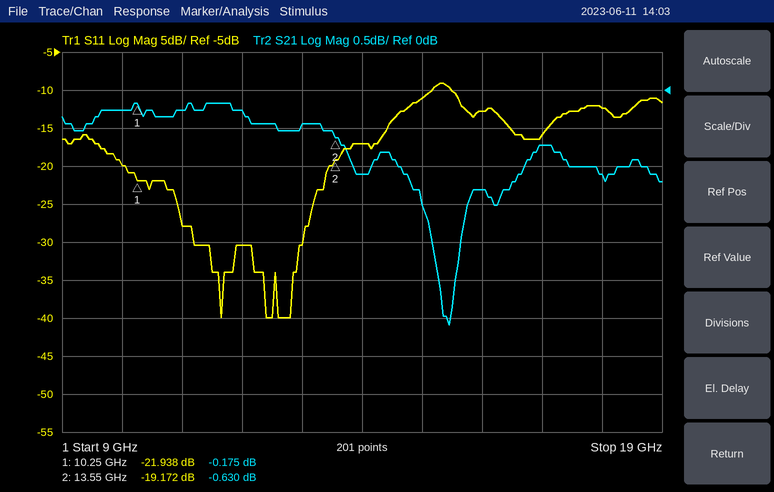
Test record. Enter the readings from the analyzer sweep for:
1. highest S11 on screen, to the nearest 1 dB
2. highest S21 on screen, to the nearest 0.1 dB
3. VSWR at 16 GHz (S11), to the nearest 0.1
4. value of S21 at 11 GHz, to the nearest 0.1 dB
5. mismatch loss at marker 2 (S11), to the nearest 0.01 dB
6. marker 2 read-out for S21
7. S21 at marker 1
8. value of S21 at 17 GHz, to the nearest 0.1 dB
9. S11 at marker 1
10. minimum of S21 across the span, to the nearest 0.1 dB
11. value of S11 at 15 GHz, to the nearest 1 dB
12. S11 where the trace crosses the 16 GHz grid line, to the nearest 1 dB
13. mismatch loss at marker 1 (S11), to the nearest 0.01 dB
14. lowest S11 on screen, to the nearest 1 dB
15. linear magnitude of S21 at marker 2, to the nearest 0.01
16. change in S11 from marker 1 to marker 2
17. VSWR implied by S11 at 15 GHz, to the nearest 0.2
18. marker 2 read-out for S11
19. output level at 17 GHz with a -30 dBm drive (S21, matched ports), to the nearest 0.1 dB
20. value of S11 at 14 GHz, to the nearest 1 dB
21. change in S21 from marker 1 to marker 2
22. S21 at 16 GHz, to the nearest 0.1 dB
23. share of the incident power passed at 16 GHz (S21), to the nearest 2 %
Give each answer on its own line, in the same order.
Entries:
-9 dB
-0.2 dB
1.6
-0.3 dB
0.05 dB
-0.630 dB
-0.175 dB
-0.7 dB
-21.938 dB
-3.1 dB
-11 dB
-13 dB
0.03 dB
-40 dB
0.93
2.766 dB
1.8
-19.172 dB
-30.7 dBm
-17 dB
-0.455 dB
-1.3 dB
74 %
